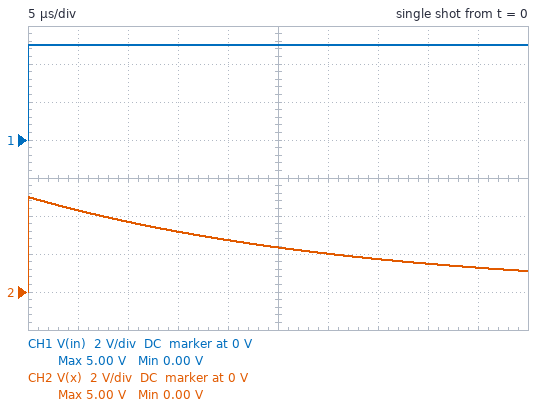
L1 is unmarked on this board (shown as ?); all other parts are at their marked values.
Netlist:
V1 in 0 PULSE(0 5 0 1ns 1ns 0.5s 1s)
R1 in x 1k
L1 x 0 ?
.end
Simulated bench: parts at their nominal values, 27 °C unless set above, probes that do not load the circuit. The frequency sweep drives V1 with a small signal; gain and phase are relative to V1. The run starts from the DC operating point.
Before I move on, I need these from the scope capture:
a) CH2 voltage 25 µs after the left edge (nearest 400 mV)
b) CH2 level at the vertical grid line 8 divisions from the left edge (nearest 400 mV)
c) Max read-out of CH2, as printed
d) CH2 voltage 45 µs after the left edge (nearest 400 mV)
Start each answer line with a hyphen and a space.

- 2.4 V
- 1.6 V
- 5.00 V
- 1.2 V
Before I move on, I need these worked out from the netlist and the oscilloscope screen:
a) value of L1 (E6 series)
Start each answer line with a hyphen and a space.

- 33 mH
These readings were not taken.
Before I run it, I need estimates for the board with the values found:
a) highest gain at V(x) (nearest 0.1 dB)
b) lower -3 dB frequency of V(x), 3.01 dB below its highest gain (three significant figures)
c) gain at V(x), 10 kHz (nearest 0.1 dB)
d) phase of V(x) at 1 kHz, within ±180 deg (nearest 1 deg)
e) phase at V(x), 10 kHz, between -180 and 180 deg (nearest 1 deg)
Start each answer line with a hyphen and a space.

- 0 dB
- 4.82 kHz
- -0.9 dB
- 78 deg
- 26 deg
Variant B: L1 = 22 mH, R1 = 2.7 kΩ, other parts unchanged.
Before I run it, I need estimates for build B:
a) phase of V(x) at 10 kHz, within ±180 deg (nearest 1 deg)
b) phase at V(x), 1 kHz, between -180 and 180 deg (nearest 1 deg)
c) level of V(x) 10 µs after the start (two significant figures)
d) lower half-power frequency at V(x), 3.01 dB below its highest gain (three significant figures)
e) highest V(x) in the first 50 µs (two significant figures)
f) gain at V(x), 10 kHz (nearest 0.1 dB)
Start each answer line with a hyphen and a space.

- 63 deg
- 87 deg
- 1.5 V
- 19.5 kHz
- 5.0 V
- -6.8 dB
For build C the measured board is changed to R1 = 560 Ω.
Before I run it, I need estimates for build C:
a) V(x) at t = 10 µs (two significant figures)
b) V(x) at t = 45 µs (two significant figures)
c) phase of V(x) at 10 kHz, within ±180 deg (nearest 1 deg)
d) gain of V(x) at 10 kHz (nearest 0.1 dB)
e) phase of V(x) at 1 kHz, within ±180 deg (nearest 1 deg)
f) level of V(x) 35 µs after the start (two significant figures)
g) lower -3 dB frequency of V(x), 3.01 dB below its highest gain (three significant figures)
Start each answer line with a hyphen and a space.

- 4.2 V
- 2.3 V
- 15 deg
- -0.3 dB
- 70 deg
- 2.8 V
- 2.70 kHz
